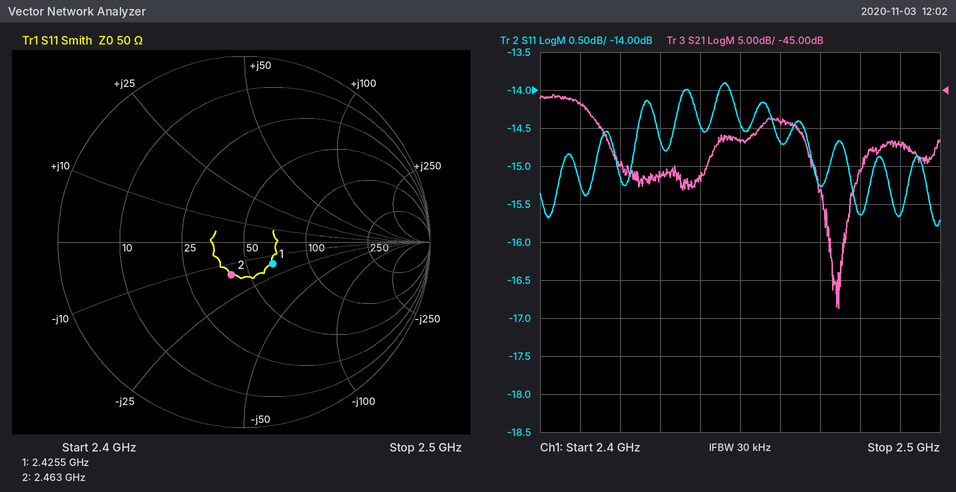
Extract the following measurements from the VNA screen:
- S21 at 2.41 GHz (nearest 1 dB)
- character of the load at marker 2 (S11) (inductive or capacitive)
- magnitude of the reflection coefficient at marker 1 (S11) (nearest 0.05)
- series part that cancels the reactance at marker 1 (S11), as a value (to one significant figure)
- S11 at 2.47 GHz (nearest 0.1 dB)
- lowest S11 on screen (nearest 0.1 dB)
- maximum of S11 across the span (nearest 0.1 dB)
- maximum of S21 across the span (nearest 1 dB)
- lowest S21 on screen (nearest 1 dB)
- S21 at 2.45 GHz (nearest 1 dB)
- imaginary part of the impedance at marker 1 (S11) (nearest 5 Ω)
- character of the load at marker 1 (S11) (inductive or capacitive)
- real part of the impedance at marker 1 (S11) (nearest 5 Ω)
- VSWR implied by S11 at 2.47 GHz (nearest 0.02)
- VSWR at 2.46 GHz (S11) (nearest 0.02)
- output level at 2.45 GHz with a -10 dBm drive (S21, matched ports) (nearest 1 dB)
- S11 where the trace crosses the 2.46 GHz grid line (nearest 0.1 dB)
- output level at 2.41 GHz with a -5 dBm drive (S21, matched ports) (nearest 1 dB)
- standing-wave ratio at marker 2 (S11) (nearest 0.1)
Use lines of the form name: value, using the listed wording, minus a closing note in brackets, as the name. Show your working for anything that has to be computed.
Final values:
S21 at 2.41 GHz: -47 dB
character of the load at marker 2 (S11): capacitive
magnitude of the reflection coefficient at marker 1 (S11): 0.20
series part that cancels the reactance at marker 1 (S11), as a value: L = 15 Ω/(2π × 2.4255 GHz) ≈ 1 nH
S11 at 2.47 GHz: -15.3 dB
lowest S11 on screen: -15.8 dB
maximum of S11 across the span: -13.9 dB
maximum of S21 across the span: -46 dB
lowest S21 on screen: -74 dB
S21 at 2.45 GHz: -52 dB
imaginary part of the impedance at marker 1 (S11): -15 Ω
character of the load at marker 1 (S11): capacitive
real part of the impedance at marker 1 (S11): 65 Ω
VSWR implied by S11 at 2.47 GHz: |Γ| = 10^(-15.3/20) = 0.1718; VSWR = (1 + 0.1718)/(1 − 0.1718) ≈ 1.41, so 1.42 to the nearest 0.02
VSWR at 2.46 GHz (S11): |Γ| = 10^(-14.7/20) = 0.1841; VSWR = (1 + 0.1841)/(1 − 0.1841) ≈ 1.45, so 1.46 to the nearest 0.02
output level at 2.45 GHz with a -10 dBm drive (S21, matched ports): -10 dBm + (-52 dB) = -62 dBm
S11 where the trace crosses the 2.46 GHz grid line: -14.7 dB
output level at 2.41 GHz with a -5 dBm drive (S21, matched ports): -5 dBm + (-47 dB) = -52 dBm
standing-wave ratio at marker 2 (S11): 1.5
